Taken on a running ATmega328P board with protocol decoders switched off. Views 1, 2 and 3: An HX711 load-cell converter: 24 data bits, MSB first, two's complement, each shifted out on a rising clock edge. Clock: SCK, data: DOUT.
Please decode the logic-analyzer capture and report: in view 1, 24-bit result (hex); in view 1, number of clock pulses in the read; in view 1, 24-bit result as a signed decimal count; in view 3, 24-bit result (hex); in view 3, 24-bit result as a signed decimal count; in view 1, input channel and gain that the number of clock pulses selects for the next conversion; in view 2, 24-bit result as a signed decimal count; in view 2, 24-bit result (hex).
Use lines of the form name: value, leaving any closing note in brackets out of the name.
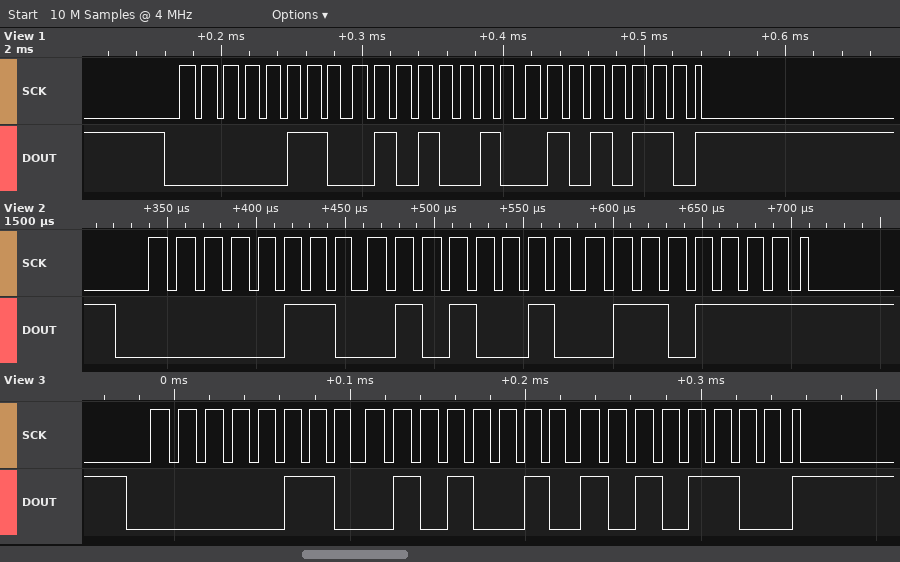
in view 1, 24-bit result: 0x065256
in view 1, number of clock pulses in the read: 25
in view 1, 24-bit result as a signed decimal count: 414294
in view 3, 24-bit result: 0x0652AC
in view 3, 24-bit result as a signed decimal count: 414380
in view 1, input channel and gain that the number of clock pulses selects for the next conversion: channel A, gain 128
in view 2, 24-bit result as a signed decimal count: 414319
in view 2, 24-bit result: 0x06526F
